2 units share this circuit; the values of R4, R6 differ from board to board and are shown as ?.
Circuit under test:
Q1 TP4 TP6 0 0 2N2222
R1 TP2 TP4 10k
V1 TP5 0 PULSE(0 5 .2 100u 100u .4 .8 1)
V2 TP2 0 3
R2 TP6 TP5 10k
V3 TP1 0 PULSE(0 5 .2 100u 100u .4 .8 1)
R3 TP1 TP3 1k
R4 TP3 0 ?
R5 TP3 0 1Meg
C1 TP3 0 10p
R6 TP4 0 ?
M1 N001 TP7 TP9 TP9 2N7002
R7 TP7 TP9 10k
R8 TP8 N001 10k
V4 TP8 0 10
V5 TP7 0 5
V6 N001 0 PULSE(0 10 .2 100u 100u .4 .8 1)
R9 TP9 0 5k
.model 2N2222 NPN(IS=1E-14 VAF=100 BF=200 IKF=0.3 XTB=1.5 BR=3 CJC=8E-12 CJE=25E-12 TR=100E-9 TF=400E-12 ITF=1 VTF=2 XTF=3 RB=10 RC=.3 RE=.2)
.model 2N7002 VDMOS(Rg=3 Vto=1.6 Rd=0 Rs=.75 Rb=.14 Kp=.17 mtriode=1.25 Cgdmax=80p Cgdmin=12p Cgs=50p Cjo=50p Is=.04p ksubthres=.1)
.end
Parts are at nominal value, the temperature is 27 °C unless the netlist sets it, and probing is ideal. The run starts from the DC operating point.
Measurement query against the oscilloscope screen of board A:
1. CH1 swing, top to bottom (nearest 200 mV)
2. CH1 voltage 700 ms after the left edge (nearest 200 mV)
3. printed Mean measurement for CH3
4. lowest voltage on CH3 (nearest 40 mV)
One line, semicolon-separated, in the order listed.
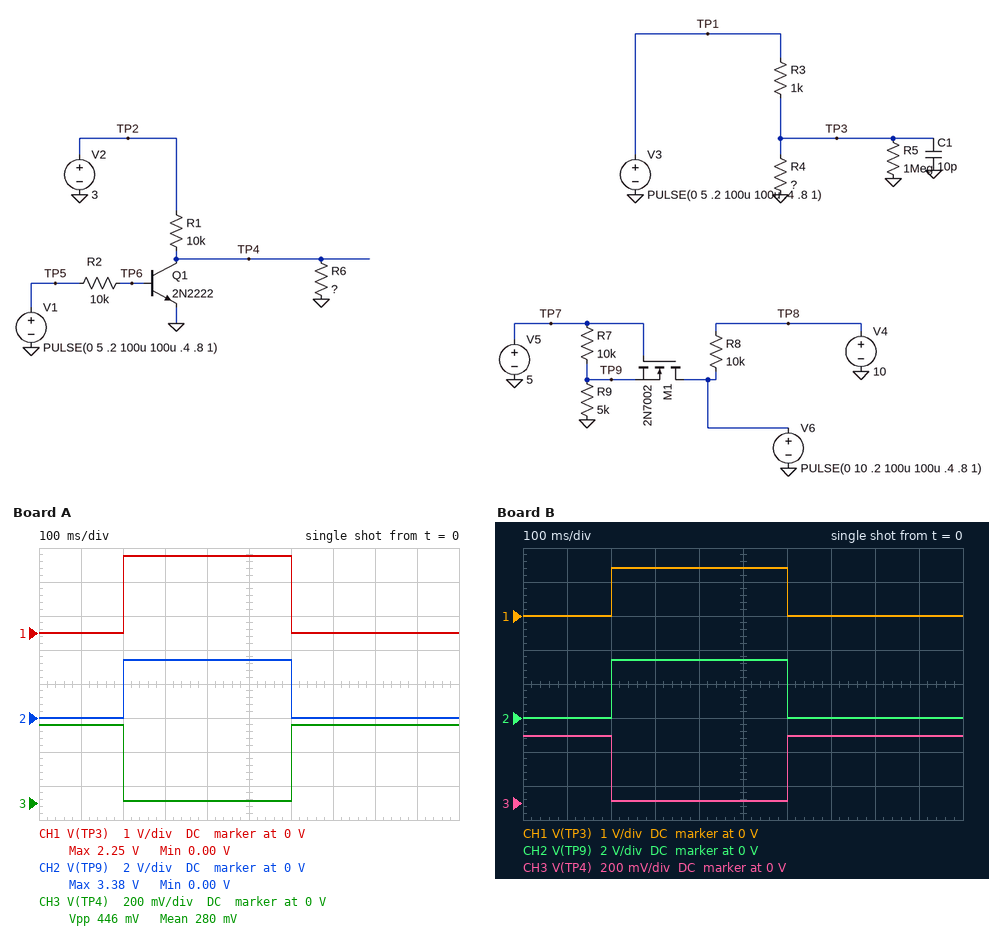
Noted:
2.2 V; 0 V; 280 mV; 0 V
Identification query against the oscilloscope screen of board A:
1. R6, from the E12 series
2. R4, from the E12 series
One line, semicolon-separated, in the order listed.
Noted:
1.8 kΩ; 820 Ω
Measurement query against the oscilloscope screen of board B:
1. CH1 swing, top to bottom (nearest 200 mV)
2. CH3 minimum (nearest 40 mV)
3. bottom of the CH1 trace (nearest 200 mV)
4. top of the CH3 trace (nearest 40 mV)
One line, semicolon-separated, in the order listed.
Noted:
1.4 V; 0 V; 0 V; 400 mV
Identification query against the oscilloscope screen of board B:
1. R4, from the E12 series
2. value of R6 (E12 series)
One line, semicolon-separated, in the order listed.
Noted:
390 Ω; 1.5 kΩ
